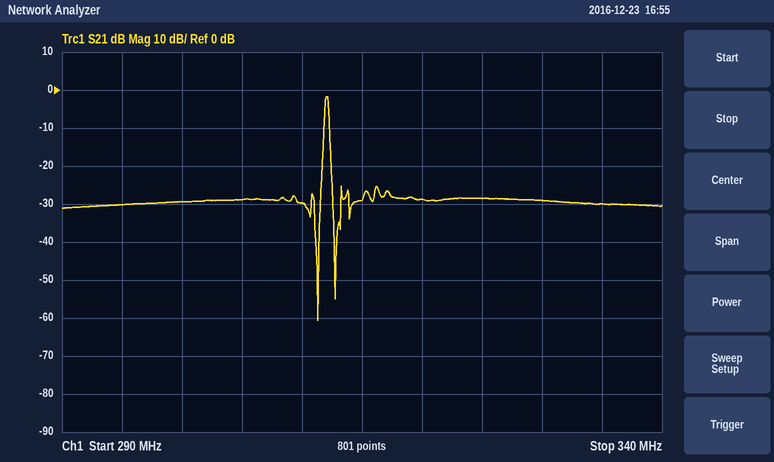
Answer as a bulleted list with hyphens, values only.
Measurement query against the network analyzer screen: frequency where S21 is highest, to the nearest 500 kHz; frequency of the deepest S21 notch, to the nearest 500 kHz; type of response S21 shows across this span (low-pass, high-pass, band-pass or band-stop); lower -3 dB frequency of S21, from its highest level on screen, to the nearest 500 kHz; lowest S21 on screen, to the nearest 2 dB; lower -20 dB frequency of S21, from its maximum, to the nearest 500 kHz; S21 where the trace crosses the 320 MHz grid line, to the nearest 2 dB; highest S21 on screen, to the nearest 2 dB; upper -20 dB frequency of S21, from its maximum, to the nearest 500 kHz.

- 312.0 MHz
- 311.5 MHz
- band-pass
- 312.0 MHz
- -60 dB
- 311.5 MHz
- -28 dB
- -2 dB
- 312.5 MHz
